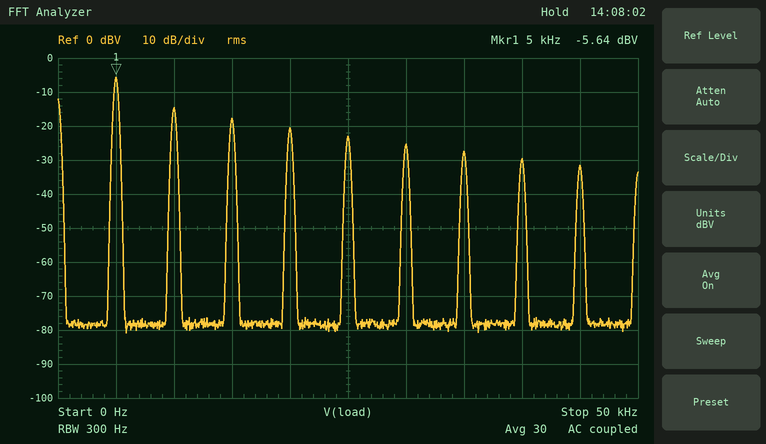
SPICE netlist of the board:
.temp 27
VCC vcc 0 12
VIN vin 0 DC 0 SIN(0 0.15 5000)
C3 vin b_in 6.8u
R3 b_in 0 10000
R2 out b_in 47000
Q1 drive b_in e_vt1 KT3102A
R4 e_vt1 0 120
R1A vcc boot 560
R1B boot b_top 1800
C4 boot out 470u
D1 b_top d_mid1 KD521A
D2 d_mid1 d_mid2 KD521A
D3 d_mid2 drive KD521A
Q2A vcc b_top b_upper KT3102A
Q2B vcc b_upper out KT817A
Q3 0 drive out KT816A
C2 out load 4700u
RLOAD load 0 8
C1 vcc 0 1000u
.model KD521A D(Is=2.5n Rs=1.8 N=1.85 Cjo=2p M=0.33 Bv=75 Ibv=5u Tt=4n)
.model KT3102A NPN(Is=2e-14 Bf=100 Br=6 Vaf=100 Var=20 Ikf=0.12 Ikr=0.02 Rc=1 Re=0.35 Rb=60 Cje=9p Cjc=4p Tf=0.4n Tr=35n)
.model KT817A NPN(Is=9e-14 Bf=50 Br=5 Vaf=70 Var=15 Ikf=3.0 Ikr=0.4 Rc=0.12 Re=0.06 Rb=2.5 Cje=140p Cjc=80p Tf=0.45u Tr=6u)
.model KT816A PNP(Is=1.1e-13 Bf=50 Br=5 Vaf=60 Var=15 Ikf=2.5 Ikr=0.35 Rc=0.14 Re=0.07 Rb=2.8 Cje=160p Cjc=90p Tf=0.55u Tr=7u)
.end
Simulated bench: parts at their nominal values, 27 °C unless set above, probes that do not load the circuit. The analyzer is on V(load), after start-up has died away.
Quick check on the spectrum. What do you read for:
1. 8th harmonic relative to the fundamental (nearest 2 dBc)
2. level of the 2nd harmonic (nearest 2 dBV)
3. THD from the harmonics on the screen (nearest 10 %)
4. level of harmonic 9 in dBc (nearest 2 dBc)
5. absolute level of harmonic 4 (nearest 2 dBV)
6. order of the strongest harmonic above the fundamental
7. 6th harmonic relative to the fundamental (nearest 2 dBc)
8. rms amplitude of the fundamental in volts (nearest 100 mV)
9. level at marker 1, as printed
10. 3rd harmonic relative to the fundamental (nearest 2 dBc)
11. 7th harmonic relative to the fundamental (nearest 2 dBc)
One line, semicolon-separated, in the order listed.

-24 dBc; -14 dBV; 50 %; -26 dBc; -20 dBV; 2; -20 dBc; 500 mV; -5.64 dBV; -12 dBc; -22 dBc
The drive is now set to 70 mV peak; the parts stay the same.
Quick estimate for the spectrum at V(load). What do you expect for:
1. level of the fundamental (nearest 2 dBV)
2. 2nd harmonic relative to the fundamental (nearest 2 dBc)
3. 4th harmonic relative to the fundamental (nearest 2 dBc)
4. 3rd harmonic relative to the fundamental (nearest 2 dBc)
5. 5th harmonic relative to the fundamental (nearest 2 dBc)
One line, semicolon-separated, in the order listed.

-14 dBV; -16 dBc; -30 dBc; -24 dBc; -36 dBc
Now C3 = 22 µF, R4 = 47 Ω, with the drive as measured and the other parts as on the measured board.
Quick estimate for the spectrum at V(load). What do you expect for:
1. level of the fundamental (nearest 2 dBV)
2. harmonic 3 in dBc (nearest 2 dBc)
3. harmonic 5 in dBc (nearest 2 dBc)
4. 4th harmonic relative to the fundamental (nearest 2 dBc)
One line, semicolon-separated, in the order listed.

2 dBV; -10 dBc; -16 dBc; -14 dBc
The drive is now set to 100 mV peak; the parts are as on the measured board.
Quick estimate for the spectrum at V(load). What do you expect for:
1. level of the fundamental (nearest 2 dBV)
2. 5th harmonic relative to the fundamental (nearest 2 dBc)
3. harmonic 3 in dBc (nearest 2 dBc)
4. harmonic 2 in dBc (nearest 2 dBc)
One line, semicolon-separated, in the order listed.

-10 dBV; -22 dBc; -16 dBc; -12 dBc
